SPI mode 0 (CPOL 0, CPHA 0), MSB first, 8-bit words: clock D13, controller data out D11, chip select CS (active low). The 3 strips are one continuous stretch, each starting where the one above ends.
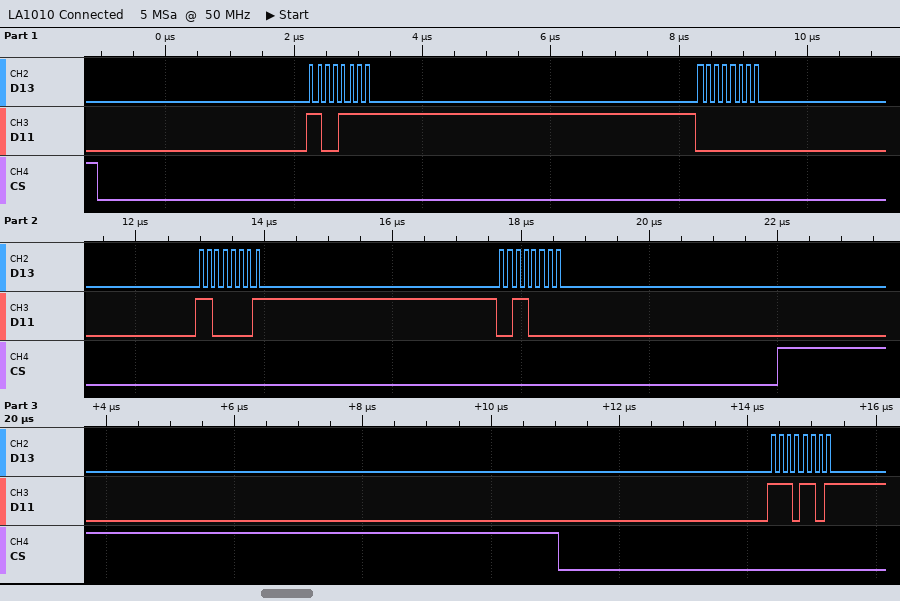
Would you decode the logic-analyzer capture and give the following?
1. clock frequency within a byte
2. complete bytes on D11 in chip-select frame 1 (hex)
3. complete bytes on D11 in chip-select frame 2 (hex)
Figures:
8 MHz
CF 00 C1 30
ED
